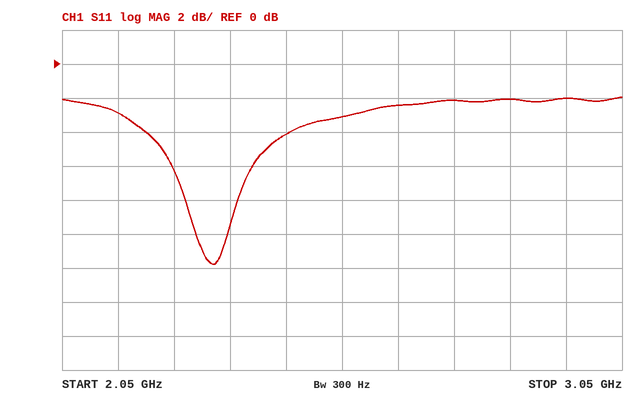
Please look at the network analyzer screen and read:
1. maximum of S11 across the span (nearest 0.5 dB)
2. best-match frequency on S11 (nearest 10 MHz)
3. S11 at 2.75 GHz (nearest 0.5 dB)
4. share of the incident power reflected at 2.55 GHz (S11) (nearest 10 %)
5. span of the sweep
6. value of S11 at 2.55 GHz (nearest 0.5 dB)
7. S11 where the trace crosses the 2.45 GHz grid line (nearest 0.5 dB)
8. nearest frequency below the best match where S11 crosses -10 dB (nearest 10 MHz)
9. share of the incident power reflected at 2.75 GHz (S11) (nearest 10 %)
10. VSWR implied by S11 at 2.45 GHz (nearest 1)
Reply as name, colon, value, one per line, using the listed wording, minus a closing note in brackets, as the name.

maximum of S11 across the span: -2.0 dB
best-match frequency on S11: 2.32 GHz
S11 at 2.75 GHz: -2.0 dB
share of the incident power reflected at 2.55 GHz (S11): 50 %
span of the sweep: 1 GHz
value of S11 at 2.55 GHz: -3.0 dB
S11 where the trace crosses the 2.45 GHz grid line: -4.0 dB
nearest frequency below the best match where S11 crosses -10 dB: 2.29 GHz
share of the incident power reflected at 2.75 GHz (S11): 60 %
VSWR implied by S11 at 2.45 GHz: 4
